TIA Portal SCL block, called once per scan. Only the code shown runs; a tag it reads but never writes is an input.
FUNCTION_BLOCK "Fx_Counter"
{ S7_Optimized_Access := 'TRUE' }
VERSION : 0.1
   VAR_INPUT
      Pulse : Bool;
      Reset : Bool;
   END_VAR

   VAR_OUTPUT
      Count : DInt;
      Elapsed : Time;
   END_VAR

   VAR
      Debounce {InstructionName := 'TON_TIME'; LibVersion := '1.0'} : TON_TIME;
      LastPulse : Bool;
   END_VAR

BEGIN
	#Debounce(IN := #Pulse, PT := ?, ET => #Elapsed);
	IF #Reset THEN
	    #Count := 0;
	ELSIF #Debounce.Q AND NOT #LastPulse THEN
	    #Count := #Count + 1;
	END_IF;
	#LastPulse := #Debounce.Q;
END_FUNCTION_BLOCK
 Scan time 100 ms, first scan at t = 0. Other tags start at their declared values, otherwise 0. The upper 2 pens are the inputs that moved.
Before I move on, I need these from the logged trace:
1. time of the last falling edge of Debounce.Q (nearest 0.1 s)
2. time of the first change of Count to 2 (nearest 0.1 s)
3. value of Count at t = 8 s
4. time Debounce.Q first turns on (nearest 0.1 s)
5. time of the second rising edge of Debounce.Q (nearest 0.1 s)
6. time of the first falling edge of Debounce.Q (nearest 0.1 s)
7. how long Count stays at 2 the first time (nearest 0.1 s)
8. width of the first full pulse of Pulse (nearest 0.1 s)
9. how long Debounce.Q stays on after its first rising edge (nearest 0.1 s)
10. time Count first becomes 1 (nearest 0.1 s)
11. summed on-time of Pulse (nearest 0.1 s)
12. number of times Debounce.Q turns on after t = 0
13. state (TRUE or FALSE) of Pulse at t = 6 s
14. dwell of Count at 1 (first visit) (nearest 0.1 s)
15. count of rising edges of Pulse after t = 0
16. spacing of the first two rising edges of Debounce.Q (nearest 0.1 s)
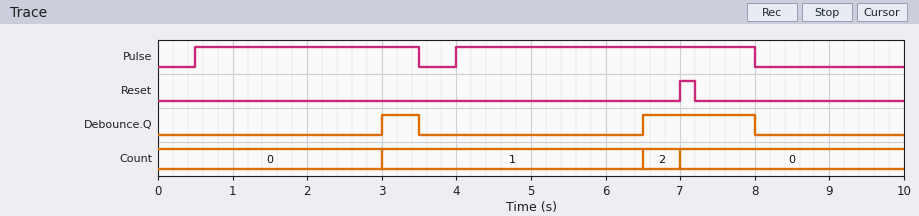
8.0 s
6.5 s
0
3.0 s
6.5 s
3.5 s
0.5 s
3.0 s
0.5 s
3.0 s
7.0 s
2
TRUE
3.5 s
2
3.5 s
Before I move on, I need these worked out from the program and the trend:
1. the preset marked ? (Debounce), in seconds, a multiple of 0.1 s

2.5 s
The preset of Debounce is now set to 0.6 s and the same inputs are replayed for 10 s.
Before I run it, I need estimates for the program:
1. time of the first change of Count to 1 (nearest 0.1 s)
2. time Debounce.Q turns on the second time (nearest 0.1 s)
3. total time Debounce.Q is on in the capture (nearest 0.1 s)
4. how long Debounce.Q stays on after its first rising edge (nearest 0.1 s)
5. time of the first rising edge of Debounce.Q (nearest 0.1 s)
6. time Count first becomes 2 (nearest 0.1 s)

1.1 s
4.6 s
5.8 s
2.4 s
1.1 s
4.6 s
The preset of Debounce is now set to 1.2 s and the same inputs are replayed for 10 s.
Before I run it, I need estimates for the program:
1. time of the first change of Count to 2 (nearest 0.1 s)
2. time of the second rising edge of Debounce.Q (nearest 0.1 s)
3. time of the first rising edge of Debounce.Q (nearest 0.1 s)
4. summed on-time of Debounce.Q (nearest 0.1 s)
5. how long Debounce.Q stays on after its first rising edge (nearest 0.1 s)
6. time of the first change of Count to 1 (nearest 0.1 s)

5.2 s
5.2 s
1.7 s
4.6 s
1.8 s
1.7 s
